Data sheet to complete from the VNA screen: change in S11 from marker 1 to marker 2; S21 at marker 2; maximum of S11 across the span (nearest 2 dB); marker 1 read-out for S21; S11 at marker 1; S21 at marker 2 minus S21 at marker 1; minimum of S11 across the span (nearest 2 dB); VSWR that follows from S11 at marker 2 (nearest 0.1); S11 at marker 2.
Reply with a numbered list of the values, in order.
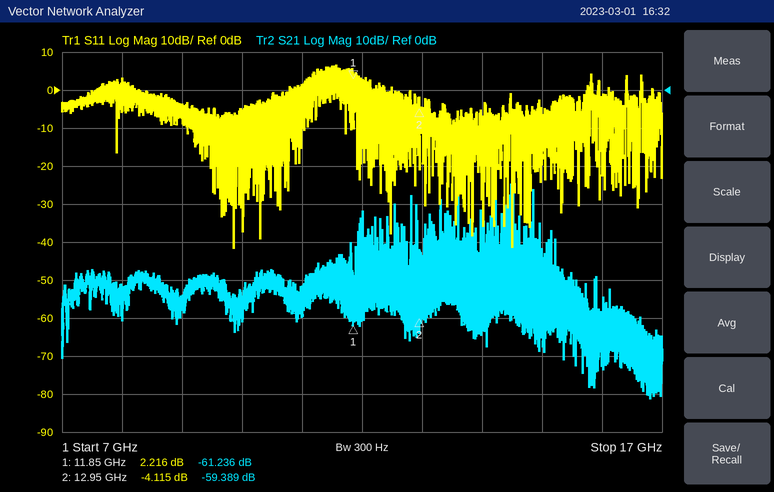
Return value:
1. -6.331 dB
2. -59.389 dB
3. 6 dB
4. -61.236 dB
5. 2.216 dB
6. 1.847 dB
7. -42 dB
8. 4.3
9. -4.115 dB
